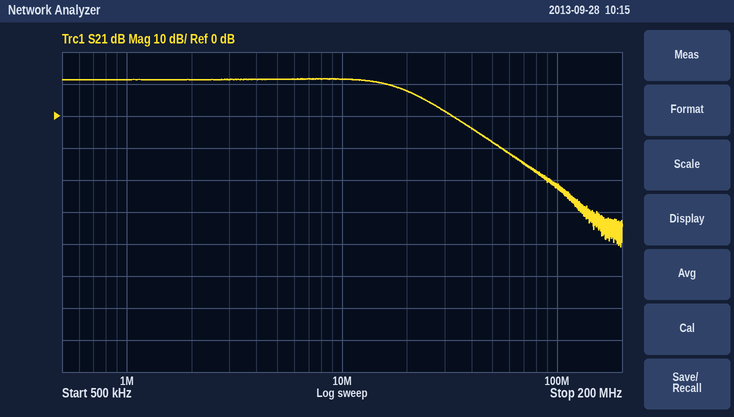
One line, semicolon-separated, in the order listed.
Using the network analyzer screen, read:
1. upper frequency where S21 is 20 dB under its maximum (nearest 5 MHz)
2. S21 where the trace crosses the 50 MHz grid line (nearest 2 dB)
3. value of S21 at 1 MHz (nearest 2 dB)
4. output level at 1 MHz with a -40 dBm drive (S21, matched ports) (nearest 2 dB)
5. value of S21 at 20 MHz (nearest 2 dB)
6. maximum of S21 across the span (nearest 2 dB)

50 MHz; -8 dB; 12 dB; -28 dBm; 8 dB; 12 dB
